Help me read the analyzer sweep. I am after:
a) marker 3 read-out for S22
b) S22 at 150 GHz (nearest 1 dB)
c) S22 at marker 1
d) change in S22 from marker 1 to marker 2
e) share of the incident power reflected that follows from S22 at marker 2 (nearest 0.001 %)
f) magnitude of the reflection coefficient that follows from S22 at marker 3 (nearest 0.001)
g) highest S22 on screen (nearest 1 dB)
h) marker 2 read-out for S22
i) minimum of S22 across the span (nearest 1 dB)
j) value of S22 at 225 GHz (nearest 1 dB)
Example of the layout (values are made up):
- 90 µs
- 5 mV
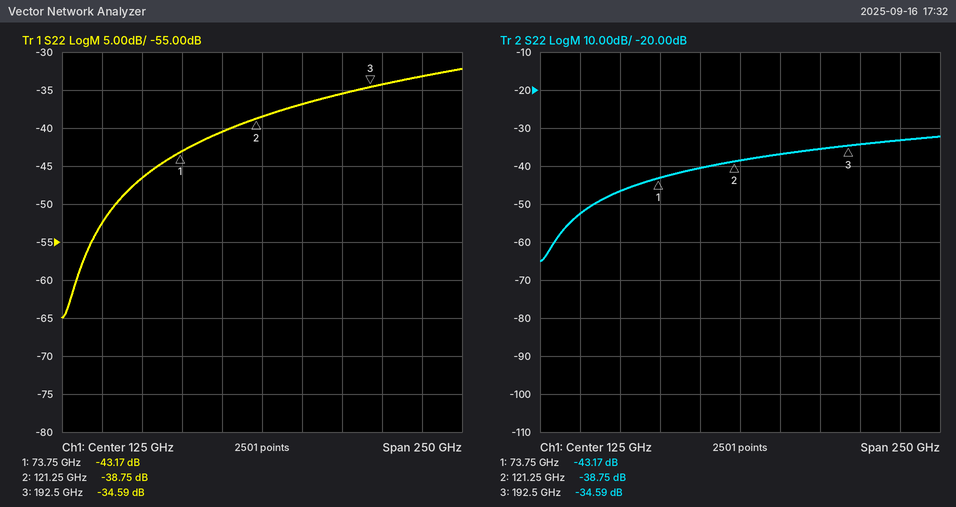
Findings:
- -34.59 dB
- -37 dB
- -43.17 dB
- 4.42 dB
- 0.013 %
- 0.019
- -32 dB
- -38.75 dB
- -65 dB
- -33 dB
